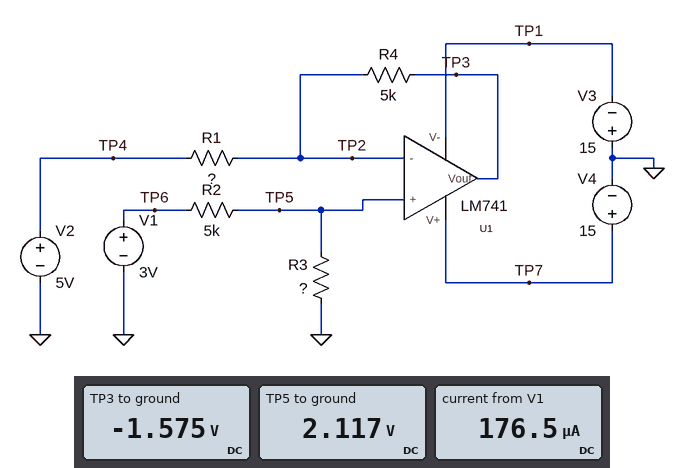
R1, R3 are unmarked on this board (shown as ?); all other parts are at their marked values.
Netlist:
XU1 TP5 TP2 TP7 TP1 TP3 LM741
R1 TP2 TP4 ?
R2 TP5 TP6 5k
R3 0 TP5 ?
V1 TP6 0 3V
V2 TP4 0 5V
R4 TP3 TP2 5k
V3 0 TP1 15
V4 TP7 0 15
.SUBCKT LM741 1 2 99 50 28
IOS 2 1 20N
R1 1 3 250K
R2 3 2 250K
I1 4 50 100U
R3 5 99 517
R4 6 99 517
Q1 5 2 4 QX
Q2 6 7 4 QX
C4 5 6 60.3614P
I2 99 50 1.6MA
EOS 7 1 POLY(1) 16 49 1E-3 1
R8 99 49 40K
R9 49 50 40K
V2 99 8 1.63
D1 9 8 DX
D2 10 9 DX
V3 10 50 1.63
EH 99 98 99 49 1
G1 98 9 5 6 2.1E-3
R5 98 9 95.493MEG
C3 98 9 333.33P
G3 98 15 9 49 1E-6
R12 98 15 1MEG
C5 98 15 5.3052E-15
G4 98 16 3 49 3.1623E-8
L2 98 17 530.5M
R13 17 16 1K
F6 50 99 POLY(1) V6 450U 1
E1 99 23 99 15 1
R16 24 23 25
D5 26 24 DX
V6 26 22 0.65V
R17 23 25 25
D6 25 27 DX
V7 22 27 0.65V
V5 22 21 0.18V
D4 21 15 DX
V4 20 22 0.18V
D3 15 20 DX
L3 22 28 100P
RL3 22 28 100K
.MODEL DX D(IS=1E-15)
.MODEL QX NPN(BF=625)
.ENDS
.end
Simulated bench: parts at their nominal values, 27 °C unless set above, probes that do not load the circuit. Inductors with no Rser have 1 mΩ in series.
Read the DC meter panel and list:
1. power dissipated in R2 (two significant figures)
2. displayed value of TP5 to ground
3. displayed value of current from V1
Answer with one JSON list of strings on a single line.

["160 µW", "2.117 V", "176.5 µA"]
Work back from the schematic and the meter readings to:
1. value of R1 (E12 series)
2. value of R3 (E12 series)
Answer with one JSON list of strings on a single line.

["3.9 kΩ", "12 kΩ"]
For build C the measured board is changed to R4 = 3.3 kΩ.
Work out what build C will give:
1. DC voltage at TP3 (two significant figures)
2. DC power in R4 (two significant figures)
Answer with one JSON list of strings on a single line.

["-320 mV", "1.8 mW"]
